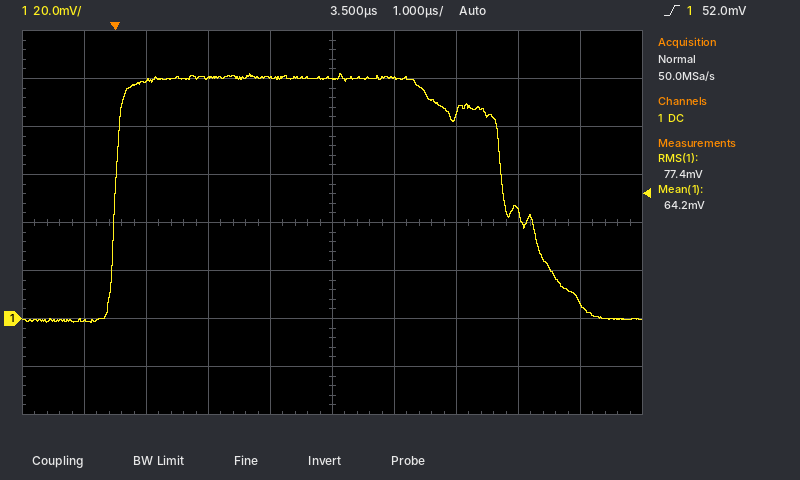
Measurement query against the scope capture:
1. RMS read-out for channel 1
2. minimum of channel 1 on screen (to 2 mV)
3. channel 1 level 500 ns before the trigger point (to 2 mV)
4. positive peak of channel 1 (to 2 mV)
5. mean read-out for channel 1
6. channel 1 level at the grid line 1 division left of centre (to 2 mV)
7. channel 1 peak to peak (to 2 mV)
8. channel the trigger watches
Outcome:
77.4 mV
-2 mV
0 mV
102 mV
64.2 mV
100 mV
104 mV
channel 1
